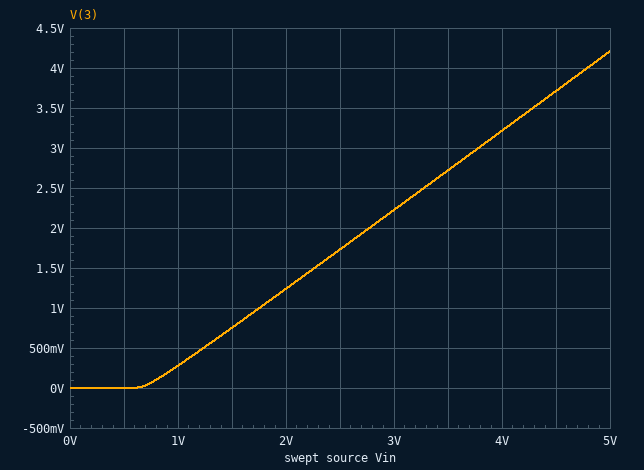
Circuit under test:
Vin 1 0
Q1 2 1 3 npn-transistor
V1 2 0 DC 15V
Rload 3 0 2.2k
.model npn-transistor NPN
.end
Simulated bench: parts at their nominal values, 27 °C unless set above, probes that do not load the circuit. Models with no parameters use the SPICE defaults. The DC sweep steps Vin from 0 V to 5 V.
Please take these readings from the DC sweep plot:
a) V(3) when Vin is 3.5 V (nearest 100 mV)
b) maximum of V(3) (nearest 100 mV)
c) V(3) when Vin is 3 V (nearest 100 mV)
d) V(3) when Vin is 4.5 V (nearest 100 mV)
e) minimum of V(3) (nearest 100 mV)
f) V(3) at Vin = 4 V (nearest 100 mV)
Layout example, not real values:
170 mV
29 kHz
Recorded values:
2.7 V
4.2 V
2.2 V
3.7 V
0 V
3.2 V
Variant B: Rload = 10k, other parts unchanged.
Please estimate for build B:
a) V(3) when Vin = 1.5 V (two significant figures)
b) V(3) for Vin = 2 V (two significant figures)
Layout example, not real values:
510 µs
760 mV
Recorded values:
790 mV
1.3 V
